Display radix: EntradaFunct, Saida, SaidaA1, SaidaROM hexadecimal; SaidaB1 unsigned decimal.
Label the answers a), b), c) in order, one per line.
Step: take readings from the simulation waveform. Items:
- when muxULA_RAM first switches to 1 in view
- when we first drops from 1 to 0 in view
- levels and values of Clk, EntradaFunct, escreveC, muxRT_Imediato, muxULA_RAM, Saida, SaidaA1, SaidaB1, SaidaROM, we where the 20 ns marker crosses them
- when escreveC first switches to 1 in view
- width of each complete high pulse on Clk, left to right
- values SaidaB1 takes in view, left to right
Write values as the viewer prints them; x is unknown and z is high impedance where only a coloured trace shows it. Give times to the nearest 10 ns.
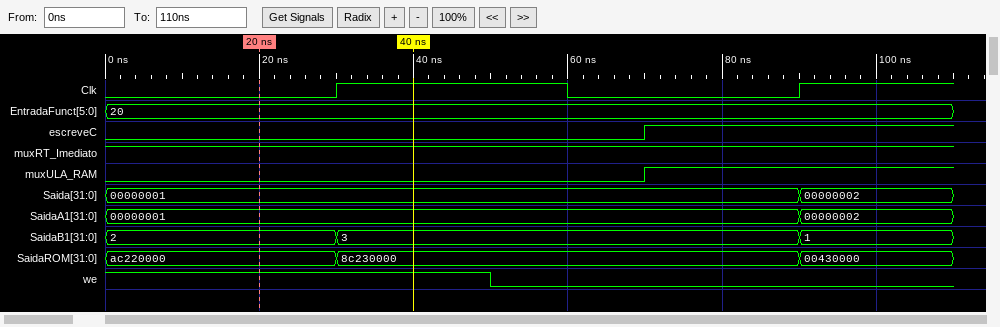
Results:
a) 70 ns
b) 50 ns
c) Clk=0, EntradaFunct=20, escreveC=0, muxRT_Imediato=1, muxULA_RAM=0, Saida=00000001, SaidaA1=00000001, SaidaB1=2, SaidaROM=ac220000, we=1
d) 70 ns
e) 30 ns
f) 2, 3, 1
